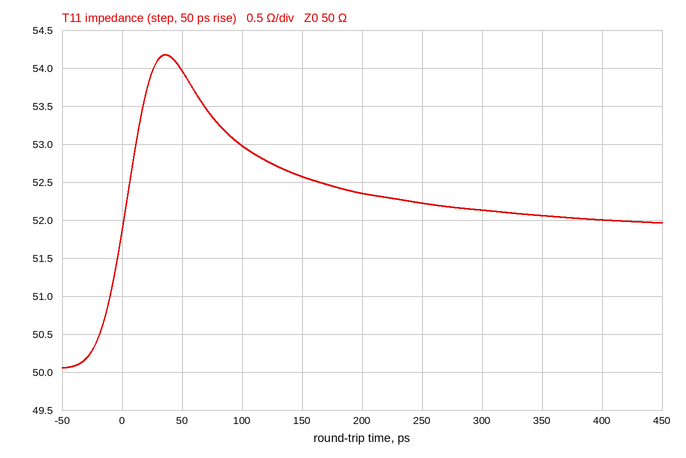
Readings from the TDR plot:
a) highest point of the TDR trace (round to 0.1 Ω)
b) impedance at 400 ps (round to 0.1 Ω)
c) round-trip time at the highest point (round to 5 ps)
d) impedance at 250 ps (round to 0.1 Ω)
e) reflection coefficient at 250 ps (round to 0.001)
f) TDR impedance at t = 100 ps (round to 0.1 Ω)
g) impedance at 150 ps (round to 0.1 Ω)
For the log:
54.2 Ω
52.0 Ω
35 ps
52.2 Ω
+0.022
53.0 Ω
52.6 Ω
